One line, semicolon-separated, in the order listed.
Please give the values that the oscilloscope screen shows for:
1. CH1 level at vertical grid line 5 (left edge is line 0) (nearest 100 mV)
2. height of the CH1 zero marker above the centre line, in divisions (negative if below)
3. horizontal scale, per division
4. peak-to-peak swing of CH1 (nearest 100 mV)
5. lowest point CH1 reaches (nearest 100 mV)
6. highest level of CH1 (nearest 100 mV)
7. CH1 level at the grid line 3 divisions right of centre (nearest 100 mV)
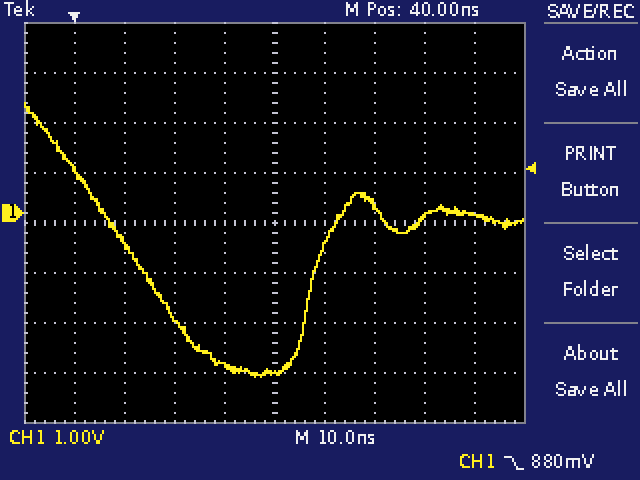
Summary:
-3.2 V; +0.2 div; 10 ns; 5.5 V; -3.3 V; 2.2 V; -100 mV
